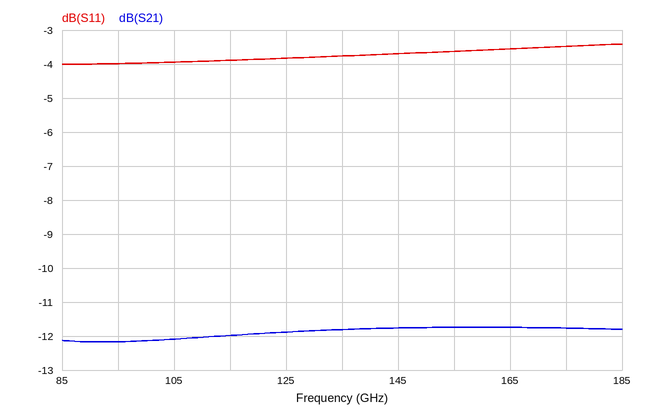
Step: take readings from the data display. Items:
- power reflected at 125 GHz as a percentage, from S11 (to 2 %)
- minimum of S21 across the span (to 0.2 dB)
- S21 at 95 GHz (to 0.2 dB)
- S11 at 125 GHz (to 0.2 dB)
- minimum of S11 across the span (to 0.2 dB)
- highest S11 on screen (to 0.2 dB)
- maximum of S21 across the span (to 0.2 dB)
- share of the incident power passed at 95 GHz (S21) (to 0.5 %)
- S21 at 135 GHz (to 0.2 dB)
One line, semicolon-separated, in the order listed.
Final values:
42 %; -12.2 dB; -12.2 dB; -3.8 dB; -4.0 dB; -3.4 dB; -11.8 dB; 6.0 %; -11.8 dB
